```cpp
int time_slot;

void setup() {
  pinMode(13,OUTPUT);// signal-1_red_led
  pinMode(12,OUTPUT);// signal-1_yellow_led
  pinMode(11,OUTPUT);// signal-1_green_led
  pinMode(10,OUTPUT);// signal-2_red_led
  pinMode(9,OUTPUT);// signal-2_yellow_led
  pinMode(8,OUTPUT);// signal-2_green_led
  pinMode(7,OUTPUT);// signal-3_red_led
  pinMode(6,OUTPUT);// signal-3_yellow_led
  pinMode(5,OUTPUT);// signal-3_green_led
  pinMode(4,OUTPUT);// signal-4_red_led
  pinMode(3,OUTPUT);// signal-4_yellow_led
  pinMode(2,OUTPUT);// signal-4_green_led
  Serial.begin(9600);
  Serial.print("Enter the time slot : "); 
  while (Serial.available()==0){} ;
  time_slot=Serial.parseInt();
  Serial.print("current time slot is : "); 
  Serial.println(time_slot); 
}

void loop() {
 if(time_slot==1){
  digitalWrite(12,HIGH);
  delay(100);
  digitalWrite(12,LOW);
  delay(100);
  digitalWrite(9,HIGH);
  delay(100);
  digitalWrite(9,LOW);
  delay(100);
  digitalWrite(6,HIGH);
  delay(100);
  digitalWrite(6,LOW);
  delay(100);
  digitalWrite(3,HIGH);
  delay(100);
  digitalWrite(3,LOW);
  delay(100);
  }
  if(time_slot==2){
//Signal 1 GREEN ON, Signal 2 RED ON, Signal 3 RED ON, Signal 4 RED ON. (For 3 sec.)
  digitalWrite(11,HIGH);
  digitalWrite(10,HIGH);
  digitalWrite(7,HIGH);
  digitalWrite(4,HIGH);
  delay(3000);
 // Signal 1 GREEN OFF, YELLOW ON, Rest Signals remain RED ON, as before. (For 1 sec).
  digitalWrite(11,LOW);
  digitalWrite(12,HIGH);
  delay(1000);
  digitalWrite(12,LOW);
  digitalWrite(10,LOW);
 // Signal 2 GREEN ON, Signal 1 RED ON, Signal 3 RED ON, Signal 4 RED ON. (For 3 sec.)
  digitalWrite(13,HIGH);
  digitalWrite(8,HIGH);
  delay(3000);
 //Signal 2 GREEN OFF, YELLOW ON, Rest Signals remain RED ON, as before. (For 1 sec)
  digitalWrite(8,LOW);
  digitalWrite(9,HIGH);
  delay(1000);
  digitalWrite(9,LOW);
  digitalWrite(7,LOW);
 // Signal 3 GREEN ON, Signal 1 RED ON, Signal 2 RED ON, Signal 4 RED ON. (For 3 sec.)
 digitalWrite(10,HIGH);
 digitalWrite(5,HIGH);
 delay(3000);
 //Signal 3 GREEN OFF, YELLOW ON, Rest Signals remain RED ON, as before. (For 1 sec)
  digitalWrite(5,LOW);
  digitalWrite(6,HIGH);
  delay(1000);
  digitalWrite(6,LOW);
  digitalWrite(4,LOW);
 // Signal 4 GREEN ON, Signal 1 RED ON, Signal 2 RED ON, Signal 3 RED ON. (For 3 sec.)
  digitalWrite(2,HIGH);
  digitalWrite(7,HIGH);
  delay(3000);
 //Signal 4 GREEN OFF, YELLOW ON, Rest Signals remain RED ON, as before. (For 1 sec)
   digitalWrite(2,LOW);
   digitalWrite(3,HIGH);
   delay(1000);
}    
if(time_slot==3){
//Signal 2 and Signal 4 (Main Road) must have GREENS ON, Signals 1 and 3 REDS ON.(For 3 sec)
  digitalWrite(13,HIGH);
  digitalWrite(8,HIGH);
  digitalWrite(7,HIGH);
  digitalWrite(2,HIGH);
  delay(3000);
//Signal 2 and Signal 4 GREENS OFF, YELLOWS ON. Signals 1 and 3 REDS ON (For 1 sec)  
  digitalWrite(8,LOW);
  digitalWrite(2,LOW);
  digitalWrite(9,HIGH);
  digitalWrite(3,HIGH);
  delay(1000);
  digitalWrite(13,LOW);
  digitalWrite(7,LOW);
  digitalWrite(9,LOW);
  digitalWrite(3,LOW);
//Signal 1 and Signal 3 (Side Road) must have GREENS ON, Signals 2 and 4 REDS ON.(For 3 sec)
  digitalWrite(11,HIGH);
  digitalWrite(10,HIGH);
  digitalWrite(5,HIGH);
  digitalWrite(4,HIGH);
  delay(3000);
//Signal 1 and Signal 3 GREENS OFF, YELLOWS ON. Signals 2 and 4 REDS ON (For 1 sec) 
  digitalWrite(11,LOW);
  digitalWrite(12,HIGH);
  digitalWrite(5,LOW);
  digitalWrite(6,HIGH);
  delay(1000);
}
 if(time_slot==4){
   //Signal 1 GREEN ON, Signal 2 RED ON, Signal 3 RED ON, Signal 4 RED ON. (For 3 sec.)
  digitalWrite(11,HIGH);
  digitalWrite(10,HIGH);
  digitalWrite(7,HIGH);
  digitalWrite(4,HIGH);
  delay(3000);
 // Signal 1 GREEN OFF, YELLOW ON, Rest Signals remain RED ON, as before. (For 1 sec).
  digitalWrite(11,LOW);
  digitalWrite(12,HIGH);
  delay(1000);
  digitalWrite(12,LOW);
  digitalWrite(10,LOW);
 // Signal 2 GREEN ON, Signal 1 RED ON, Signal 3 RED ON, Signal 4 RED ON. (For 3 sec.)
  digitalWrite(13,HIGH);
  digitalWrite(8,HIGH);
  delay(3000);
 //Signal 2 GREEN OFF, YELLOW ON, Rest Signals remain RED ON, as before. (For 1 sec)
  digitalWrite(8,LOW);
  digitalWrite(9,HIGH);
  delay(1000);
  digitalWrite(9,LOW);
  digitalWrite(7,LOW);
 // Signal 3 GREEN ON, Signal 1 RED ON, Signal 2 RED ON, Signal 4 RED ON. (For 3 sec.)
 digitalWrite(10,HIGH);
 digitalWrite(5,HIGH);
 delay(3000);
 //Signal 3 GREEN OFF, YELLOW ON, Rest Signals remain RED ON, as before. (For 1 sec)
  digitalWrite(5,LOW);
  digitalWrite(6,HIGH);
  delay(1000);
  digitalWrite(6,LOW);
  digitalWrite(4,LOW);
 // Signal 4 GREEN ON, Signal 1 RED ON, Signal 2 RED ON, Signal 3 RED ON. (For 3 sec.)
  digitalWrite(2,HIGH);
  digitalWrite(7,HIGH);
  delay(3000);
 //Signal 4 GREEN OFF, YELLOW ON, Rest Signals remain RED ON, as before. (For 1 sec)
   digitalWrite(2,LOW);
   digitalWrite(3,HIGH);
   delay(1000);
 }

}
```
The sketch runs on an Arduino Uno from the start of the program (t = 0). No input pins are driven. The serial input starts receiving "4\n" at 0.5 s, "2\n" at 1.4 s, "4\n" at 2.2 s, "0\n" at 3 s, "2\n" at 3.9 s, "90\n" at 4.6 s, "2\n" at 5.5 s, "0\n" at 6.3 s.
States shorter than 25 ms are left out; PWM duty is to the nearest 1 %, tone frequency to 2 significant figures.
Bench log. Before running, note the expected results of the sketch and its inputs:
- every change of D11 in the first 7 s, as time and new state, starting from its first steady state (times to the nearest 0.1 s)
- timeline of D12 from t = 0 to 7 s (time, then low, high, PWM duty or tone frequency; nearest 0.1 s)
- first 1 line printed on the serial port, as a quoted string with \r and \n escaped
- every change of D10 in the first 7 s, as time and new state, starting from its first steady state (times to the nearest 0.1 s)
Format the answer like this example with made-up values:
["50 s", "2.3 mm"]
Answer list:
["0 s low; 0.5 s high; 3.5 s low", "0 s low; 3.5 s high; 4.5 s low", "\"Enter the time slot : current time slot is : 4\\r\\n\"", "0 s low; 0.5 s high; 4.5 s low"]
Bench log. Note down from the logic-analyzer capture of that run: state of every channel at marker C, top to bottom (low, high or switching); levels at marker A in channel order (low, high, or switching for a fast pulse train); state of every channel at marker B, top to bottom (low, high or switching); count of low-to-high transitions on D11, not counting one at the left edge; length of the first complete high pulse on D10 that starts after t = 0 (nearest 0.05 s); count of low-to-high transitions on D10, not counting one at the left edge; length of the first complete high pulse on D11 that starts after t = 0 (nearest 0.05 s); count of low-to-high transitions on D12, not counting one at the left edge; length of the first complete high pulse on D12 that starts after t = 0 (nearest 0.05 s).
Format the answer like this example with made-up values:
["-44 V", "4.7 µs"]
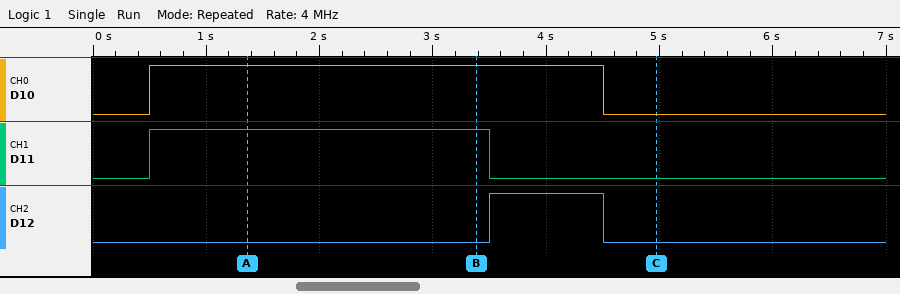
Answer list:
["D10 low, D11 low, D12 low", "D10 high, D11 high, D12 low", "D10 high, D11 high, D12 low", "1", "4.00 s", "1", "3.00 s", "1", "1.00 s"]
